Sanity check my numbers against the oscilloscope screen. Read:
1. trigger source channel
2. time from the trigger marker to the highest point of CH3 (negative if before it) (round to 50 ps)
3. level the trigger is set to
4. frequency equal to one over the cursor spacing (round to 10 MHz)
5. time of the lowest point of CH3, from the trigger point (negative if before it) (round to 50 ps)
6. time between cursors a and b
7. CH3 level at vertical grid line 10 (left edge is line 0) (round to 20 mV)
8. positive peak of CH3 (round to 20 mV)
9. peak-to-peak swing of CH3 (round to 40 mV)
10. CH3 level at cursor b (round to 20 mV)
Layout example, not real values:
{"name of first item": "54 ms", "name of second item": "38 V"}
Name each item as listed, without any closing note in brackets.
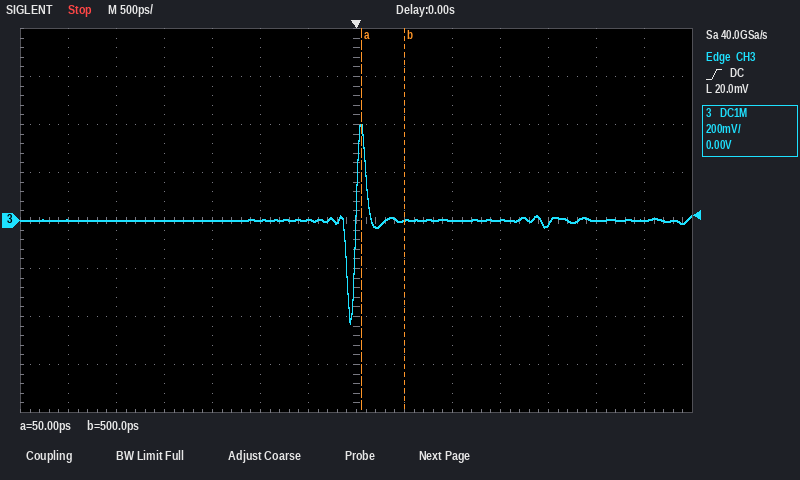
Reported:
{"trigger source channel": "CH3", "time from the trigger marker to the highest point of CH3 (negative if before it)": "+50 ps", "level the trigger is set to": "20.0 mV", "frequency equal to one over the cursor spacing": "2.22 GHz", "time of the lowest point of CH3, from the trigger point (negative if before it)": "-50 ps", "time between cursors a and b": "450 ps", "CH3 level at vertical grid line 10 (left edge is line 0)": "0 mV", "positive peak of CH3": "400 mV", "peak-to-peak swing of CH3": "840 mV", "CH3 level at cursor b": "0 mV"}
